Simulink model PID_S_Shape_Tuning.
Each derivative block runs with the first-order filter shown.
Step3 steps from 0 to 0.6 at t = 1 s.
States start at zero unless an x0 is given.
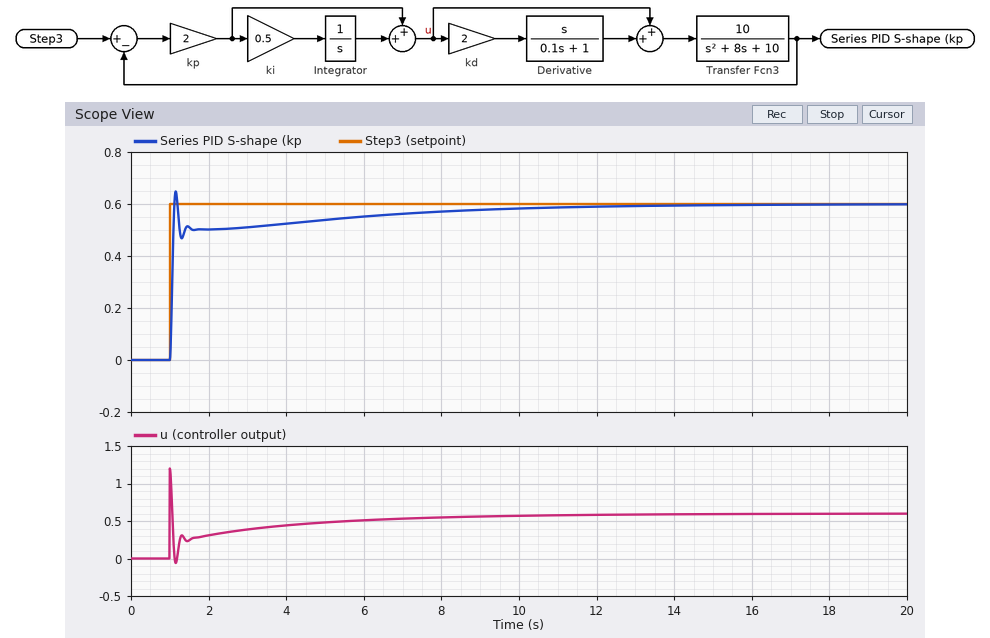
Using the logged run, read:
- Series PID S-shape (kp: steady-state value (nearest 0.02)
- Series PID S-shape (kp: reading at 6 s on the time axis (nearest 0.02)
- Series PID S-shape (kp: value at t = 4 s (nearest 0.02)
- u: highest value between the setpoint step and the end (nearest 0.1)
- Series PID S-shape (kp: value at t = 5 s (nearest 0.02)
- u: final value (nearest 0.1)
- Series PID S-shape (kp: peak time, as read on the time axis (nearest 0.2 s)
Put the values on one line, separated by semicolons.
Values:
0.60; 0.56; 0.52; 1.2; 0.54; 0.6; 1.2 s
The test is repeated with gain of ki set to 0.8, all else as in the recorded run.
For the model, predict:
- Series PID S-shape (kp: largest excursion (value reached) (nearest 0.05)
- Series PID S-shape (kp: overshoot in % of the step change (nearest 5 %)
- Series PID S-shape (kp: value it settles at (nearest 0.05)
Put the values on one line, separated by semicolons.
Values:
0.65; 10 %; 0.60
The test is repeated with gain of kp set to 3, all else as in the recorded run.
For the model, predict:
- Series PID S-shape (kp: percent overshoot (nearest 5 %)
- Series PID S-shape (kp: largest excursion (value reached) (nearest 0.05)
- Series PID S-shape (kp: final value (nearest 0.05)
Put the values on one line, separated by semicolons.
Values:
20 %; 0.70; 0.60
